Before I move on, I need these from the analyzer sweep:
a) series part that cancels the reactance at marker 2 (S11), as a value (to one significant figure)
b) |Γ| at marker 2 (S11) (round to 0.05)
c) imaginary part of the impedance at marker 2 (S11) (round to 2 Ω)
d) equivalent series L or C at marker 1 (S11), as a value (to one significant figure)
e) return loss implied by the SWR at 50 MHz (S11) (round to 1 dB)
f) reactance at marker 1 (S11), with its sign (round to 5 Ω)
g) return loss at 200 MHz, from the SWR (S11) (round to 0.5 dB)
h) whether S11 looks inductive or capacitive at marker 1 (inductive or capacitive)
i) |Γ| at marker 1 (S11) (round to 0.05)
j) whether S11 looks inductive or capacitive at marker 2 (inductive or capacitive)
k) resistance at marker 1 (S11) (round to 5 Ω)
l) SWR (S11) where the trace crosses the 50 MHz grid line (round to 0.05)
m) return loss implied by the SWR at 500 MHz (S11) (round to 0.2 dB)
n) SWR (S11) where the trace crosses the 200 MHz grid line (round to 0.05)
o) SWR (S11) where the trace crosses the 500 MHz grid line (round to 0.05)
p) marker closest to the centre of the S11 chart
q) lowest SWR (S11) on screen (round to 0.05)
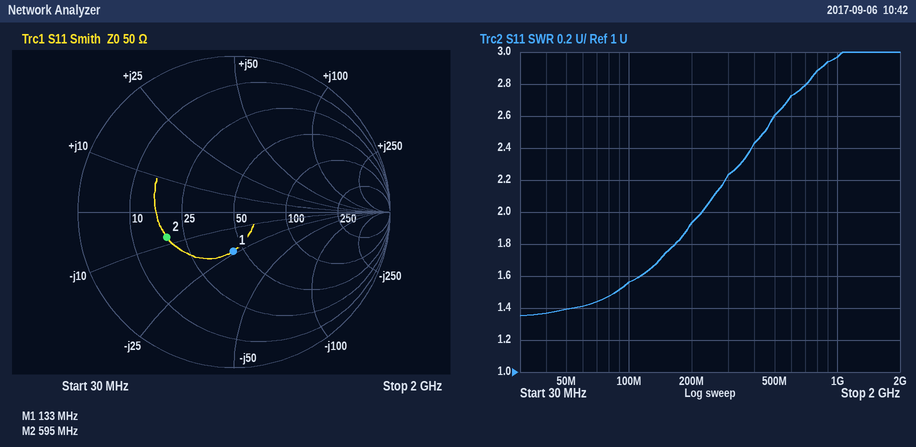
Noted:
2 nH
0.45
-8 Ω
50 pF
16 dB
-25 Ω
10.0 dB
capacitive
0.25
capacitive
45 Ω
1.40
7.0 dB
1.95
2.60
marker 1
1.35
